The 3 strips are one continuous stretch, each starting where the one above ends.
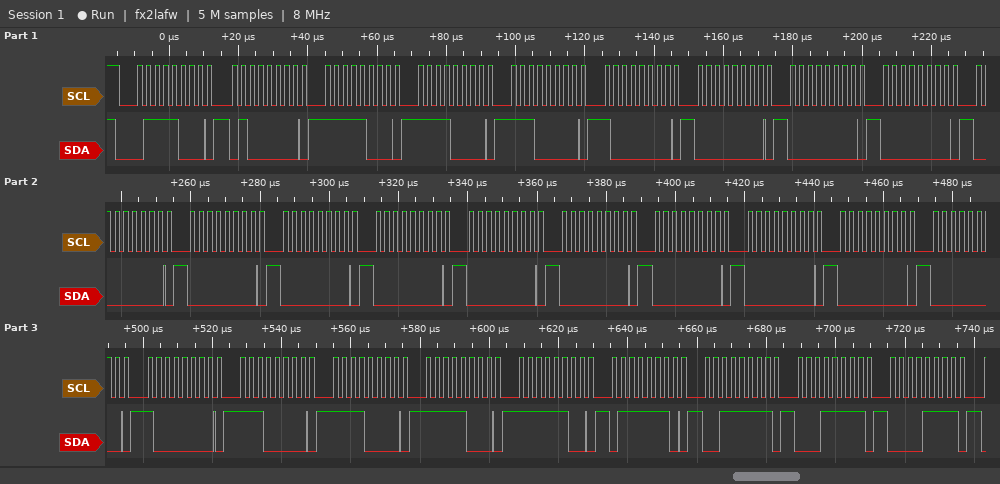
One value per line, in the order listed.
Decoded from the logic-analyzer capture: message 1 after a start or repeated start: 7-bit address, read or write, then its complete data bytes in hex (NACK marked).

0x3C write: 40 F8 F0 E0 80 00 00 00 00 00 00 00 00 00 00 00 00 00 80 E0 F0 F8 FC 7E 3F 1F 0F
